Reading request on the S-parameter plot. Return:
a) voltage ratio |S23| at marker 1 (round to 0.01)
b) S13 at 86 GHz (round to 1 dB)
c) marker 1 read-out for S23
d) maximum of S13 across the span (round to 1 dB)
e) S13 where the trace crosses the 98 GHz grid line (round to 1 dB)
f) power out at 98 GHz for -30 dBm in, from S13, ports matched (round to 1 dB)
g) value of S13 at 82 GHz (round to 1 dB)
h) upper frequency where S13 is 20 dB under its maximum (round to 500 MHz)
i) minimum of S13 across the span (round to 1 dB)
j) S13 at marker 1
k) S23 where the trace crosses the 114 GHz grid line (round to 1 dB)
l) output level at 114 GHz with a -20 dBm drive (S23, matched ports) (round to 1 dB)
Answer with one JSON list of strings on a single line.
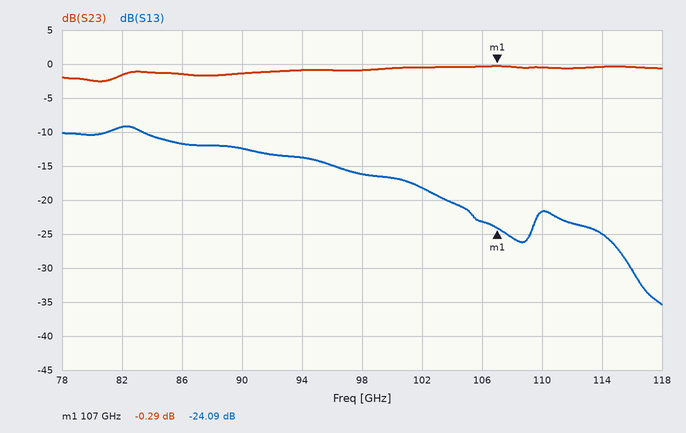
["0.97", "-12 dB", "-0.29 dB", "-9 dB", "-16 dB", "-46 dBm", "-9 dB", "115.5 GHz", "-35 dB", "-24.09 dB", "0 dB", "-20 dBm"]
